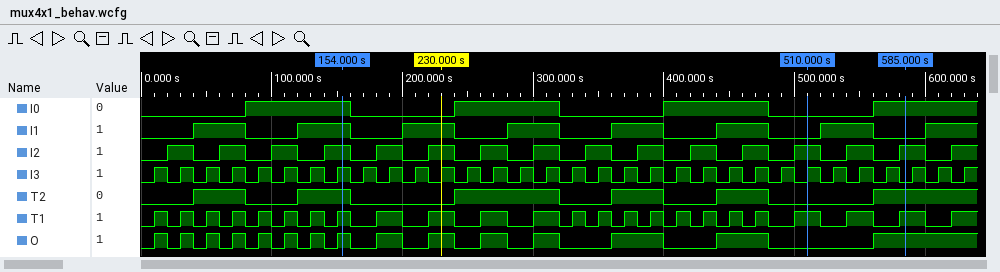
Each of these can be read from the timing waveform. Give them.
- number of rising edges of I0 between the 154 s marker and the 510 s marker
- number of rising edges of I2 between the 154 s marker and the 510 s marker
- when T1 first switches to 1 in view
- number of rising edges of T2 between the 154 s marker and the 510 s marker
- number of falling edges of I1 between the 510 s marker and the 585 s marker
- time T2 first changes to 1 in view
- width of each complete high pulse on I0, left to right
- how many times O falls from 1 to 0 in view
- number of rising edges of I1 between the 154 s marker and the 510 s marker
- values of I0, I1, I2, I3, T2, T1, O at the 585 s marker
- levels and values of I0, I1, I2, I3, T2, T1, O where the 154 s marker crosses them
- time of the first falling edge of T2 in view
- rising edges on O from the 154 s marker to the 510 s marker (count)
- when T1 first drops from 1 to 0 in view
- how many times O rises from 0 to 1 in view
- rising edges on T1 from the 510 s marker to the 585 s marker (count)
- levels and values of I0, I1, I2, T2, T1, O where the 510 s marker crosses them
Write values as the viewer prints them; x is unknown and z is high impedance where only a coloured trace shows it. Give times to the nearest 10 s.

2
9
10 s
3
1
40 s
80 s, 80 s, 80 s
14
4
I0=1, I1=0, I2=1, I3=0, T2=1, T1=1, O=1
I0=1, I1=1, I2=1, I3=1, T2=1, T1=1, O=1
80 s
6
20 s
15
2
I0=0, I1=0, I2=1, T2=0, T1=1, O=0
